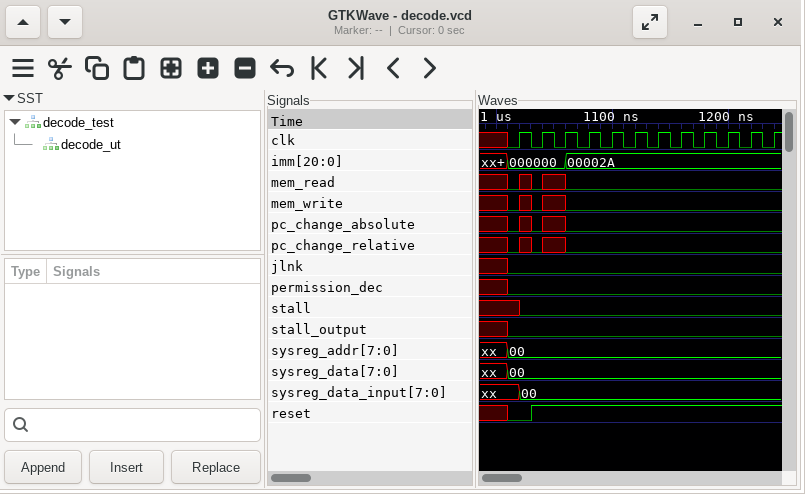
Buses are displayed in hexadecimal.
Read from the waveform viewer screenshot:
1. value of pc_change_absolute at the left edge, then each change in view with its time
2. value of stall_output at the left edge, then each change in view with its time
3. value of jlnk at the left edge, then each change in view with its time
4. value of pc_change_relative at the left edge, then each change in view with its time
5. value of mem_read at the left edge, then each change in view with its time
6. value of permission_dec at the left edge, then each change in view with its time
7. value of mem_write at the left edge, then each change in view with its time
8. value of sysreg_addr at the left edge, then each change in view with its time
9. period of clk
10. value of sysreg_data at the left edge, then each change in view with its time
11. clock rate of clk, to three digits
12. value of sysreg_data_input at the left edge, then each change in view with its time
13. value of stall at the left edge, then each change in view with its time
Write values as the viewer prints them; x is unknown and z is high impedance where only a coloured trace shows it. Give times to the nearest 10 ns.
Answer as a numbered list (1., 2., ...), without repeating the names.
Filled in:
1. x, 0 at 1010 ns, x at 1020 ns, 0 at 1030 ns, x at 1040 ns, 0 at 1060 ns
2. x, 0 at 1010 ns
3. x, 0 at 1010 ns
4. x, 0 at 1010 ns, x at 1020 ns, 0 at 1030 ns, x at 1040 ns, 0 at 1060 ns
5. x, 0 at 1010 ns, x at 1020 ns, 0 at 1030 ns, x at 1040 ns, 0 at 1060 ns
6. x, 0 at 1010 ns
7. x, 0 at 1010 ns, x at 1020 ns, 0 at 1030 ns, x at 1040 ns, 0 at 1060 ns
8. xx, 00 at 1010 ns
9. 20 ns
10. xx, 00 at 1010 ns
11. 50.0 MHz
12. xx, 00 at 1020 ns
13. x, 0 at 1020 ns
